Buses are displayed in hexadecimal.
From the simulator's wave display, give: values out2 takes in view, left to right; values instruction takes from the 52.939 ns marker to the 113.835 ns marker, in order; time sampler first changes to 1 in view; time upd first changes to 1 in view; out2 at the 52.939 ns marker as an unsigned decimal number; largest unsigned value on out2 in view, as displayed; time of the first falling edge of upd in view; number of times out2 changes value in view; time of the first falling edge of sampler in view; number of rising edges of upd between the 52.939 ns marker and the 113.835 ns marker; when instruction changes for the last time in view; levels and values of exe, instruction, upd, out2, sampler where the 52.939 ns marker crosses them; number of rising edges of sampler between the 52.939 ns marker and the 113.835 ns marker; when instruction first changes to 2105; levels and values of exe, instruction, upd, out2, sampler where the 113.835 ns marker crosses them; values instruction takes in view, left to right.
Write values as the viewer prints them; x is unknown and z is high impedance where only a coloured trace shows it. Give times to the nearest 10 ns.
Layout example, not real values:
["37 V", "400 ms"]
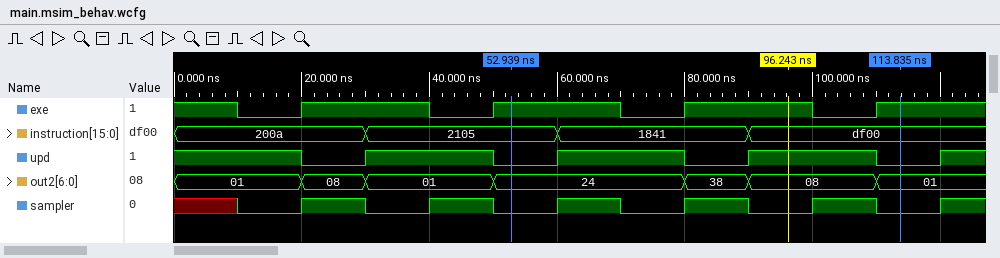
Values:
["01, 08, 01, 24, 38, 08, 01", "2105, 1841, df00", "20 ns", "30 ns", "36", "38", "20 ns", "6", "30 ns", "2", "90 ns", "exe=1, instruction=2105, upd=0, out2=24, sampler=0", "3", "30 ns", "exe=1, instruction=df00, upd=0, out2=01, sampler=0", "200a, 2105, 1841, df00"]
